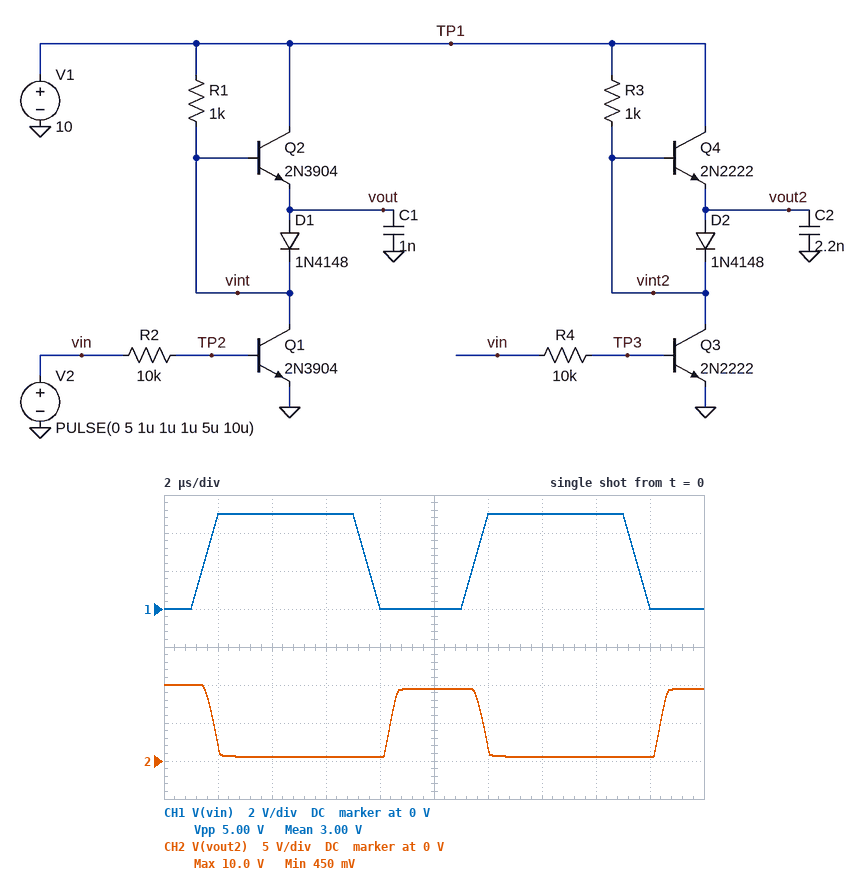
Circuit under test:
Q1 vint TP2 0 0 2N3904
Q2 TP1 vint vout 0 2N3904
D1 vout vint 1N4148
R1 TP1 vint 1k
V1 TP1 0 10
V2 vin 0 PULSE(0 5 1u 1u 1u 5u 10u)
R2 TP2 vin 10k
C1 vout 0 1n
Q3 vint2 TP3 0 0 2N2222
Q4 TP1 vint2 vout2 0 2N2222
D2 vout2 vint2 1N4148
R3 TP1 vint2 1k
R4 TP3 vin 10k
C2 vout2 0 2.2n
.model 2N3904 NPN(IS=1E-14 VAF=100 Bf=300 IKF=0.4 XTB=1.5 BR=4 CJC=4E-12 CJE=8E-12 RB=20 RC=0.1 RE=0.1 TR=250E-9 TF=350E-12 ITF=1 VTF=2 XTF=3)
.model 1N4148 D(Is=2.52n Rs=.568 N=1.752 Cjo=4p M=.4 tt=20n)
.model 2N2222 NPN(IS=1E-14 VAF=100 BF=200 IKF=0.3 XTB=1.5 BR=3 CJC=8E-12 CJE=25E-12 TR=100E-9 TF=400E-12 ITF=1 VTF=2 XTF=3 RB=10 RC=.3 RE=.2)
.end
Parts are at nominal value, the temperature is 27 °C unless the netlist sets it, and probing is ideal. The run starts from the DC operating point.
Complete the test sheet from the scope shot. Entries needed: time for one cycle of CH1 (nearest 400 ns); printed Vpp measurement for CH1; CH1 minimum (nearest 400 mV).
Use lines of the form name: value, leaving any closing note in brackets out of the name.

time for one cycle of CH1: 10.0 µs
printed Vpp measurement for CH1: 5.00 V
CH1 minimum: 0 V
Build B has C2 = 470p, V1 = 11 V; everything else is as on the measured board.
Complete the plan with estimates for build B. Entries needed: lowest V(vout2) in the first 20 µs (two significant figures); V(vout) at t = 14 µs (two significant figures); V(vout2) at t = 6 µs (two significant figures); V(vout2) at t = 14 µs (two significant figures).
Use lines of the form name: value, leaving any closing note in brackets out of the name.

lowest V(vout2) in the first 20 µs: 410 mV
V(vout) at t = 14 µs: 480 mV
V(vout2) at t = 6 µs: 420 mV
V(vout2) at t = 14 µs: 450 mV
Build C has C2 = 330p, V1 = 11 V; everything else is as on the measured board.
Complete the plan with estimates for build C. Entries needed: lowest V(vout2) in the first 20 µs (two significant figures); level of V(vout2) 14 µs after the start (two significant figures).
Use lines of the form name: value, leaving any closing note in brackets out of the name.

lowest V(vout2) in the first 20 µs: 390 mV
level of V(vout2) 14 µs after the start: 440 mV
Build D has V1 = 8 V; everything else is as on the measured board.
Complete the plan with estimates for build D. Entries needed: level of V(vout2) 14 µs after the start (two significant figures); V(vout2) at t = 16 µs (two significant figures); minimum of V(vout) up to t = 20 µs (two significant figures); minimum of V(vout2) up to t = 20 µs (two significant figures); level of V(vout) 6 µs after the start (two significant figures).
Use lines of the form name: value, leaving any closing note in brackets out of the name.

level of V(vout2) 14 µs after the start: 510 mV
V(vout2) at t = 16 µs: 480 mV
minimum of V(vout) up to t = 20 µs: 410 mV
minimum of V(vout2) up to t = 20 µs: 460 mV
level of V(vout) 6 µs after the start: 440 mV
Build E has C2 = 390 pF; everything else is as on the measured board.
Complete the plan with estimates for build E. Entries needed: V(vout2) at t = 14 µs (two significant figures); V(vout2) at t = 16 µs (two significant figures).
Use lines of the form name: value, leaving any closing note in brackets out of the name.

V(vout2) at t = 14 µs: 440 mV
V(vout2) at t = 16 µs: 410 mV
